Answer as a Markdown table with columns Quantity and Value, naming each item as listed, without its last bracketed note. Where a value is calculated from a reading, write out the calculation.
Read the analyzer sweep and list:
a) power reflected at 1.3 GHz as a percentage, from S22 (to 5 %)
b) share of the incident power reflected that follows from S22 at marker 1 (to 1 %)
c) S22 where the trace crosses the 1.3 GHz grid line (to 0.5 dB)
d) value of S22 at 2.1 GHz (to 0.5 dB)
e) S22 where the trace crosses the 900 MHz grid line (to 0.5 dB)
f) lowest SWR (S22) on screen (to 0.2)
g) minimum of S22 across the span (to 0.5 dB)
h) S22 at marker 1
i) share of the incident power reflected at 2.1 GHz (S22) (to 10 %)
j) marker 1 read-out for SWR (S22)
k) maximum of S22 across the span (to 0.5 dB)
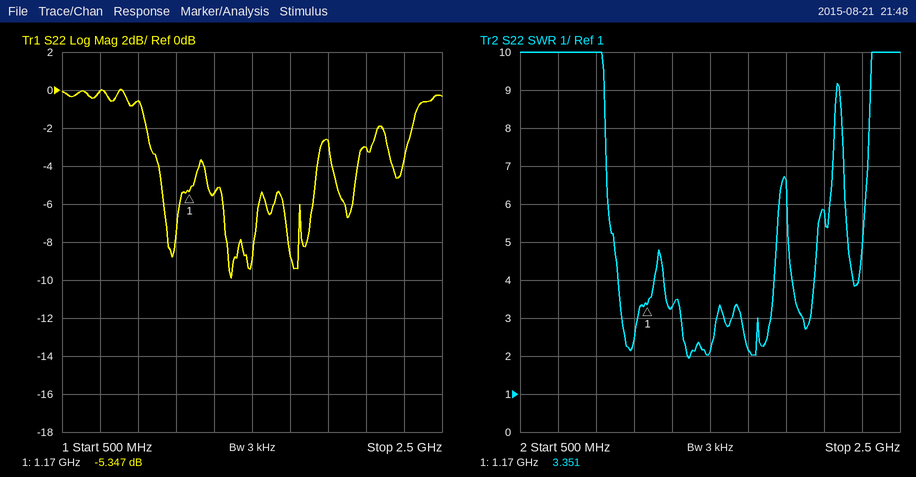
| Quantity | Value |
|---|---|
| power reflected at 1.3 GHz as a percentage, from S22 | 10^(-5.5/10) ≈ 28.2 %, so 30 % to the nearest 5 % |
| share of the incident power reflected that follows from S22 at marker 1 | 10^(-5.347/10) ≈ 29 % |
| S22 where the trace crosses the 1.3 GHz grid line | -5.5 dB |
| value of S22 at 2.1 GHz | -3.0 dB |
| S22 where the trace crosses the 900 MHz grid line | -0.5 dB |
| lowest SWR (S22) on screen | 2.0 |
| minimum of S22 across the span | -10.0 dB |
| S22 at marker 1 | -5.347 dB |
| share of the incident power reflected at 2.1 GHz (S22) | 10^(-3/10) ≈ 50 % |
| marker 1 read-out for SWR | 3.351 |
| maximum of S22 across the span | 0.0 dB |
